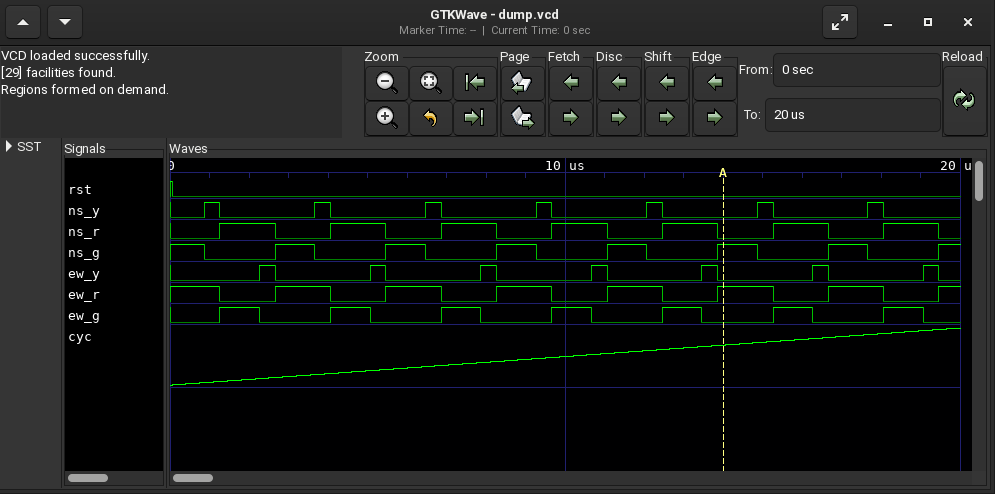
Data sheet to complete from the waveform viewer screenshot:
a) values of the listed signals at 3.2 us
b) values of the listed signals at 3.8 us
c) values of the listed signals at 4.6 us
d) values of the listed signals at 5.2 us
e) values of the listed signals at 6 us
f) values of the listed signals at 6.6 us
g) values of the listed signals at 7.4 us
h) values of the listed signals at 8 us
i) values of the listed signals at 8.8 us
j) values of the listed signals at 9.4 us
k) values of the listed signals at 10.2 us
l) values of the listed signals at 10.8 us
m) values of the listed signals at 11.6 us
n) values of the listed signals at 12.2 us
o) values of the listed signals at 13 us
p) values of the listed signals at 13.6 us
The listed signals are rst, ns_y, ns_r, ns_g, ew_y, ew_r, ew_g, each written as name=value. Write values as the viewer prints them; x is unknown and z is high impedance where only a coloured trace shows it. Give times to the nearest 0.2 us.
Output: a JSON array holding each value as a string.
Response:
["rst=0, ns_y=0, ns_r=0, ns_g=1, ew_y=0, ew_r=1, ew_g=0", "rst=0, ns_y=1, ns_r=0, ns_g=0, ew_y=0, ew_r=1, ew_g=0", "rst=0, ns_y=0, ns_r=1, ns_g=0, ew_y=0, ew_r=0, ew_g=1", "rst=0, ns_y=0, ns_r=1, ns_g=0, ew_y=1, ew_r=0, ew_g=0", "rst=0, ns_y=0, ns_r=0, ns_g=1, ew_y=0, ew_r=1, ew_g=0", "rst=0, ns_y=1, ns_r=0, ns_g=0, ew_y=0, ew_r=1, ew_g=0", "rst=0, ns_y=0, ns_r=1, ns_g=0, ew_y=0, ew_r=0, ew_g=1", "rst=0, ns_y=0, ns_r=1, ns_g=0, ew_y=1, ew_r=0, ew_g=0", "rst=0, ns_y=0, ns_r=0, ns_g=1, ew_y=0, ew_r=1, ew_g=0", "rst=0, ns_y=1, ns_r=0, ns_g=0, ew_y=0, ew_r=1, ew_g=0", "rst=0, ns_y=0, ns_r=1, ns_g=0, ew_y=0, ew_r=0, ew_g=1", "rst=0, ns_y=0, ns_r=1, ns_g=0, ew_y=1, ew_r=0, ew_g=0", "rst=0, ns_y=0, ns_r=0, ns_g=1, ew_y=0, ew_r=1, ew_g=0", "rst=0, ns_y=1, ns_r=0, ns_g=0, ew_y=0, ew_r=1, ew_g=0", "rst=0, ns_y=0, ns_r=1, ns_g=0, ew_y=0, ew_r=0, ew_g=1", "rst=0, ns_y=0, ns_r=1, ns_g=0, ew_y=1, ew_r=0, ew_g=0"]
